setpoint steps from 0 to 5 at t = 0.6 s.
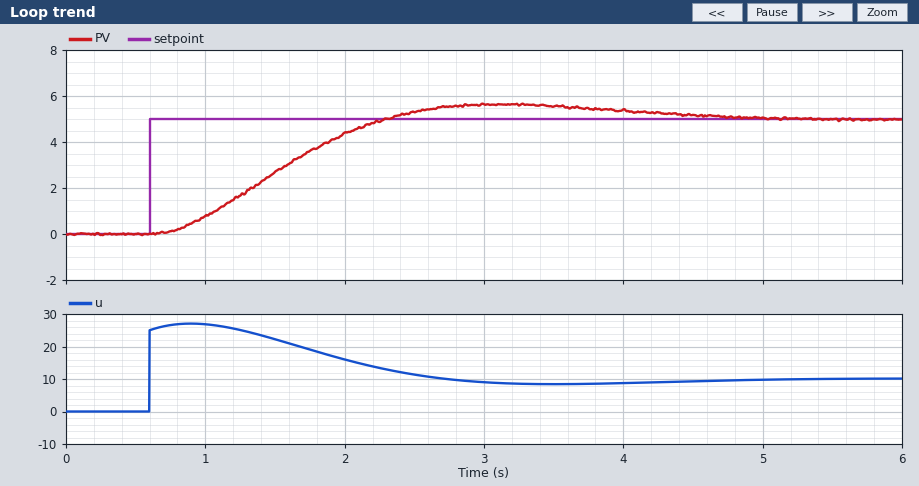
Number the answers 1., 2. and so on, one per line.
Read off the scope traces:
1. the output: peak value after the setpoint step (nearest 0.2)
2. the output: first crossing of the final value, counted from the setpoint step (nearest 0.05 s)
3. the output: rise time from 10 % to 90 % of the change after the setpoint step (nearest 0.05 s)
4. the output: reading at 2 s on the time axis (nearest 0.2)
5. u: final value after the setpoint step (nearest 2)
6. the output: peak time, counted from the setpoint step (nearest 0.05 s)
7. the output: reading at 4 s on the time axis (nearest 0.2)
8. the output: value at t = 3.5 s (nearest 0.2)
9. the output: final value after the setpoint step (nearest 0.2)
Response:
1. 5.6
2. 1.70 s
3. 1.15 s
4. 4.4
5. 10
6. 2.50 s
7. 5.4
8. 5.6
9. 5.0
